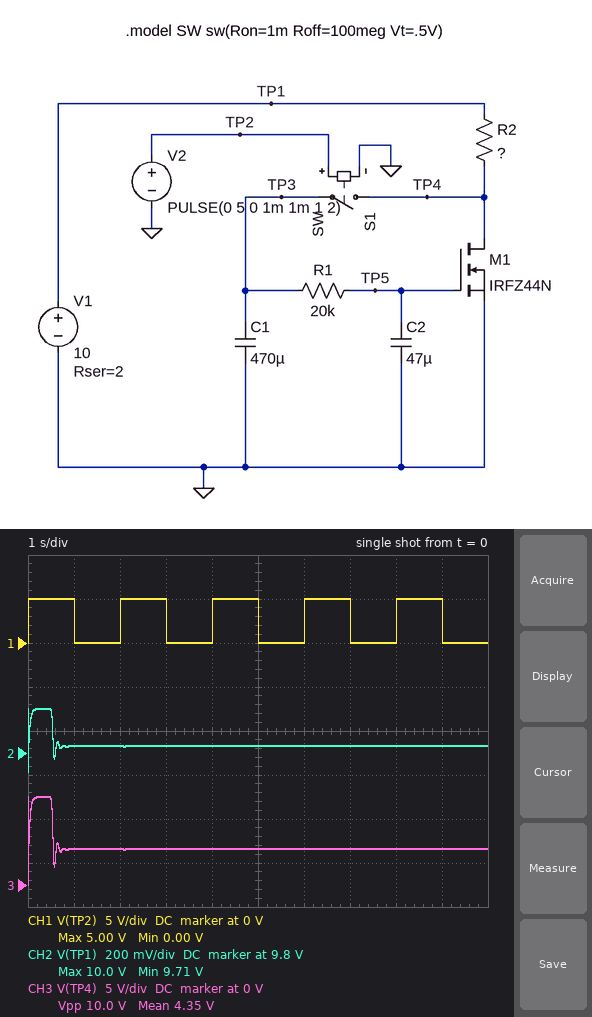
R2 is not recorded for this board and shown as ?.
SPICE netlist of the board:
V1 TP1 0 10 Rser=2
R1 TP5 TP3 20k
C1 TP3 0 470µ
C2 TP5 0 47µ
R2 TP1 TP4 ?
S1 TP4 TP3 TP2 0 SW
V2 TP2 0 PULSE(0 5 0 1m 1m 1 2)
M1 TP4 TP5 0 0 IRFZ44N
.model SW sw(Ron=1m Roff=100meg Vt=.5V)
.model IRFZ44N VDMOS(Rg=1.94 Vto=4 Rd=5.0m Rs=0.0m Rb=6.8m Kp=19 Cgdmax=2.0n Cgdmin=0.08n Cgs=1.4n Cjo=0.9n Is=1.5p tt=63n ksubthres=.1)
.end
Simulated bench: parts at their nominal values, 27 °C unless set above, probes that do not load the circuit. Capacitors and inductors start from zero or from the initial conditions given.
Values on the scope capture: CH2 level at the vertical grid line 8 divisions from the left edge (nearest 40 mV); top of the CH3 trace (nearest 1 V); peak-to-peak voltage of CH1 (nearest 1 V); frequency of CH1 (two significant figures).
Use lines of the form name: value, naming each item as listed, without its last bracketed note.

CH2 level at the vertical grid line 8 divisions from the left edge: 9.84 V
top of the CH3 trace: 10 V
peak-to-peak voltage of CH1: 5 V
frequency of CH1: 500 mHz
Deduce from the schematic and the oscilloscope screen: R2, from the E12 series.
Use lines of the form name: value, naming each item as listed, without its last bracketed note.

R2, from the E12 series: 68 Ω
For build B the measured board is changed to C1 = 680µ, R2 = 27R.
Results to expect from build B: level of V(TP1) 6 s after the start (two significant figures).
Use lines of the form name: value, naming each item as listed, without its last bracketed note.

level of V(TP1) 6 s after the start: 9.6 V
